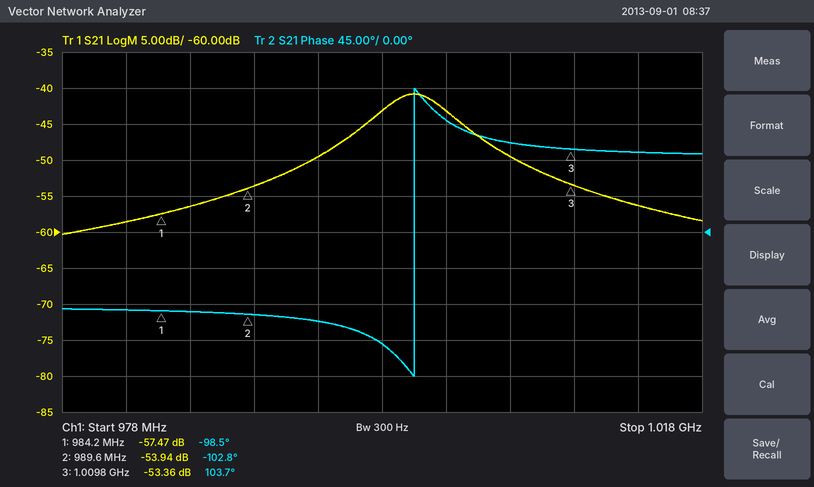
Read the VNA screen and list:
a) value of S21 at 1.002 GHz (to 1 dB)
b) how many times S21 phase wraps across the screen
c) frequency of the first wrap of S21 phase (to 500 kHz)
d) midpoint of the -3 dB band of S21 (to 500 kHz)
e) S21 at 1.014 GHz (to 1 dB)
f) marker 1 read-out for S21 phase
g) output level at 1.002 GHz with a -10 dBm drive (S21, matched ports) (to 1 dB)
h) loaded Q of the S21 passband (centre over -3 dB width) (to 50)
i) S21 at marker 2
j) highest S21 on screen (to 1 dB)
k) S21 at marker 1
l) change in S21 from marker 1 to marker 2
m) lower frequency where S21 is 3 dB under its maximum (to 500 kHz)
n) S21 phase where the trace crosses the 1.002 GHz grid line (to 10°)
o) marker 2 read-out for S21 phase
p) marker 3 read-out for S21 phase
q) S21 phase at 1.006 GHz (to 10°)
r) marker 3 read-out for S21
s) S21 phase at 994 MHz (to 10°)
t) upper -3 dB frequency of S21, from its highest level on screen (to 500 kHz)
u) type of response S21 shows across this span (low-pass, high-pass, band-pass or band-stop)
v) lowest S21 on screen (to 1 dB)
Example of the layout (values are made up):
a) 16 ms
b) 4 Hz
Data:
a) -43 dB
b) 1
c) 1.0000 GHz
d) 1.0000 GHz
e) -56 dB
f) -98.5°
g) -53 dBm
h) 200
i) -53.94 dB
j) -41 dB
k) -57.47 dB
l) 3.53 dB
m) 997.5 MHz
n) 140°
o) -102.8°
p) 103.7°
q) 110°
r) -53.36 dB
s) -110°
t) 1.0025 GHz
u) band-pass
v) -60 dB
